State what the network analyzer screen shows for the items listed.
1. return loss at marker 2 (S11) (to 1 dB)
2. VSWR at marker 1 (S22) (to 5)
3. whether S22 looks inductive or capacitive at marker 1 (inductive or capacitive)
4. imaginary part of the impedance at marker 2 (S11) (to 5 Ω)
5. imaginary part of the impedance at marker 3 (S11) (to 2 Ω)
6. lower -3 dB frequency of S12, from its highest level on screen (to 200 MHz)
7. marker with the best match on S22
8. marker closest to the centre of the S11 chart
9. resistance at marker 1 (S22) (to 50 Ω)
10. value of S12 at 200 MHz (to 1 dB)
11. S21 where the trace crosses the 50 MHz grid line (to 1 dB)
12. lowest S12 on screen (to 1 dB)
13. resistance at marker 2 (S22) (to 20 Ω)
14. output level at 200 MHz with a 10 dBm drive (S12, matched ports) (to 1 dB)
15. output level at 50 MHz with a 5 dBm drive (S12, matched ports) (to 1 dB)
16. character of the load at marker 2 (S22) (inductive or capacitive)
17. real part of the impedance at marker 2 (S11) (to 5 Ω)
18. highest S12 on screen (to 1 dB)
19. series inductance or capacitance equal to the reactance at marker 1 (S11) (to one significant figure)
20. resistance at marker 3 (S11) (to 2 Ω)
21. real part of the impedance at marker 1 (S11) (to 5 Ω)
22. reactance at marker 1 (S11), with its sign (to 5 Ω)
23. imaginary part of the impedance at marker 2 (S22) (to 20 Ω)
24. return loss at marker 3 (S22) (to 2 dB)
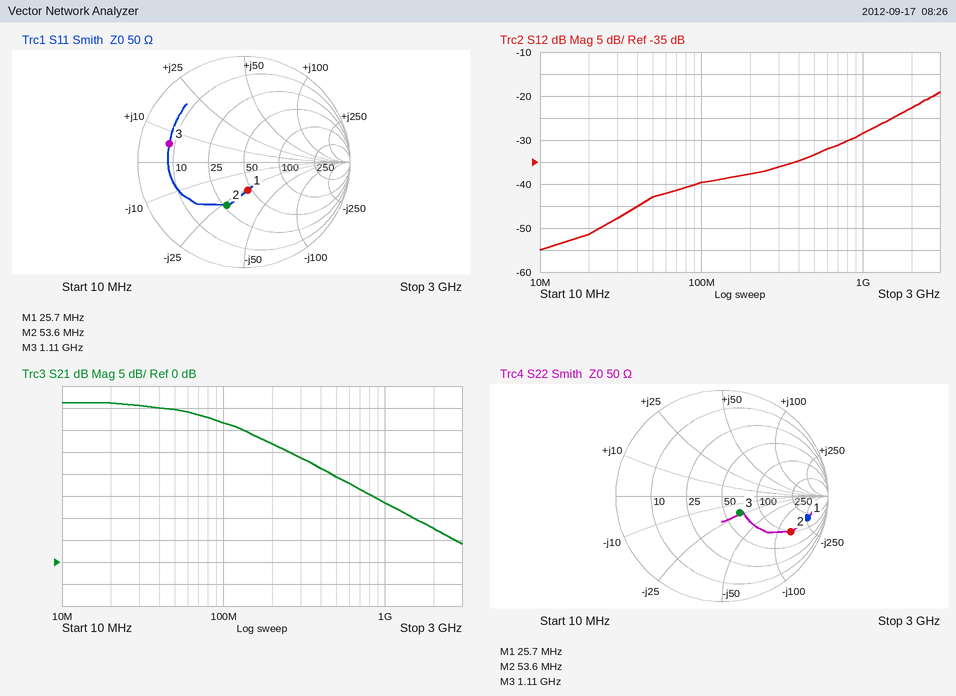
7 dB
10
capacitive
-25 Ω
+6 Ω
2.2 GHz
marker 3
marker 1
200 Ω
-38 dB
35 dB
-55 dB
100 Ω
-28 dBm
-38 dBm
capacitive
25 Ω
-19 dB
200 pF
8 Ω
45 Ω
-25 Ω
-140 Ω
12 dB
